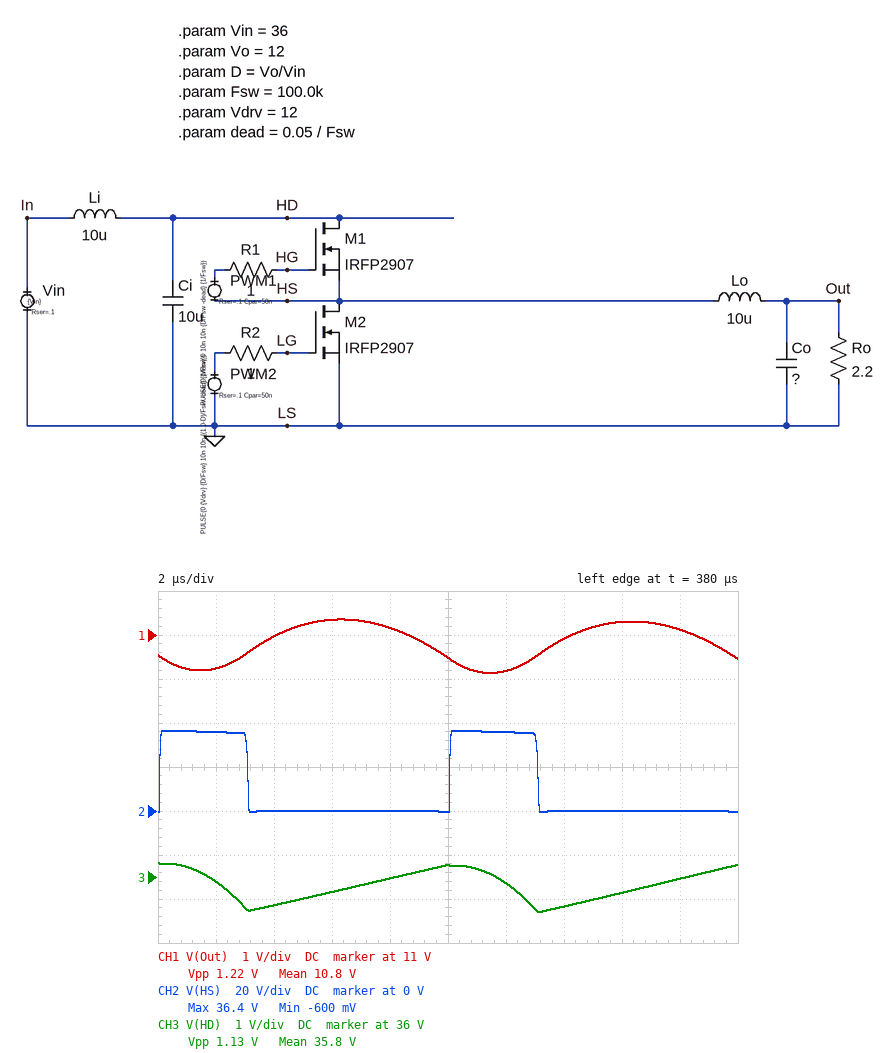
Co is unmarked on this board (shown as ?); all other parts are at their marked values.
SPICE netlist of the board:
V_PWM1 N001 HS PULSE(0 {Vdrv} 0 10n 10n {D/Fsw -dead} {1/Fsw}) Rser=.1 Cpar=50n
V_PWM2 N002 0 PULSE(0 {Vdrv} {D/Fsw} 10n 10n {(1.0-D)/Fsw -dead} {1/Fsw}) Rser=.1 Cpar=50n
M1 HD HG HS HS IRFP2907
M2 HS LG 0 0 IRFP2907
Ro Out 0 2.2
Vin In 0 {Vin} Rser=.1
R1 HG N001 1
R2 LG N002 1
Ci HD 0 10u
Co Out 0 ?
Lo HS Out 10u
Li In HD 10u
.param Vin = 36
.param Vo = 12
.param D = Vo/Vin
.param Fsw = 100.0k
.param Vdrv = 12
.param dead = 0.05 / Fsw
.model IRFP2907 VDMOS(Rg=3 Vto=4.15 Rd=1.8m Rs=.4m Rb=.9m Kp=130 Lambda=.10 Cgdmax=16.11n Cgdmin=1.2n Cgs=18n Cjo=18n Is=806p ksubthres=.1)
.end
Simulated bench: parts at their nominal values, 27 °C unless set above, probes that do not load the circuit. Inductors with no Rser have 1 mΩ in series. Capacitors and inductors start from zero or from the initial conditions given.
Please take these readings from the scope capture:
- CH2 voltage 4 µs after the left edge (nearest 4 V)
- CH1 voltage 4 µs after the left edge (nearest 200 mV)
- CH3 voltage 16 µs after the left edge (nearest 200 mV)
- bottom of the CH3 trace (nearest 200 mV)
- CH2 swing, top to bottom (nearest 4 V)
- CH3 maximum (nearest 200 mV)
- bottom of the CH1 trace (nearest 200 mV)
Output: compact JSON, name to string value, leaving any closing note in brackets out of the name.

{"CH2 voltage 4 µs after the left edge": "0 V", "CH1 voltage 4 µs after the left edge": "11.0 V", "CH3 voltage 16 µs after the left edge": "35.6 V", "bottom of the CH3 trace": "35.2 V", "CH2 swing, top to bottom": "36 V", "CH3 maximum": "36.4 V", "bottom of the CH1 trace": "10.2 V"}
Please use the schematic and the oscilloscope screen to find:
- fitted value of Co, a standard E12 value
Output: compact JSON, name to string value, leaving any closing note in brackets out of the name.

{"fitted value of Co, a standard E12 value": "8.2 µF"}
